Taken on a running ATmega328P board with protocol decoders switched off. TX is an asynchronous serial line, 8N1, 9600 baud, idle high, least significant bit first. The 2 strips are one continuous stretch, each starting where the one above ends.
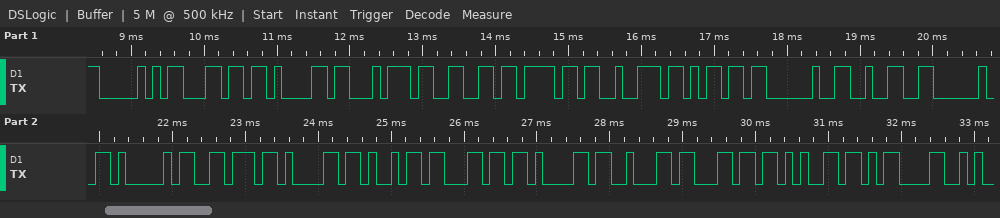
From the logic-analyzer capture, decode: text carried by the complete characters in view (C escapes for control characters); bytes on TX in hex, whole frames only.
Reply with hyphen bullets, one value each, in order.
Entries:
- "Platform 2 Available\r"
- 50 6C 61 74 66 6F 72 6D 20 32 20 41 76 61 69 6C 61 62 6C 65 0D
